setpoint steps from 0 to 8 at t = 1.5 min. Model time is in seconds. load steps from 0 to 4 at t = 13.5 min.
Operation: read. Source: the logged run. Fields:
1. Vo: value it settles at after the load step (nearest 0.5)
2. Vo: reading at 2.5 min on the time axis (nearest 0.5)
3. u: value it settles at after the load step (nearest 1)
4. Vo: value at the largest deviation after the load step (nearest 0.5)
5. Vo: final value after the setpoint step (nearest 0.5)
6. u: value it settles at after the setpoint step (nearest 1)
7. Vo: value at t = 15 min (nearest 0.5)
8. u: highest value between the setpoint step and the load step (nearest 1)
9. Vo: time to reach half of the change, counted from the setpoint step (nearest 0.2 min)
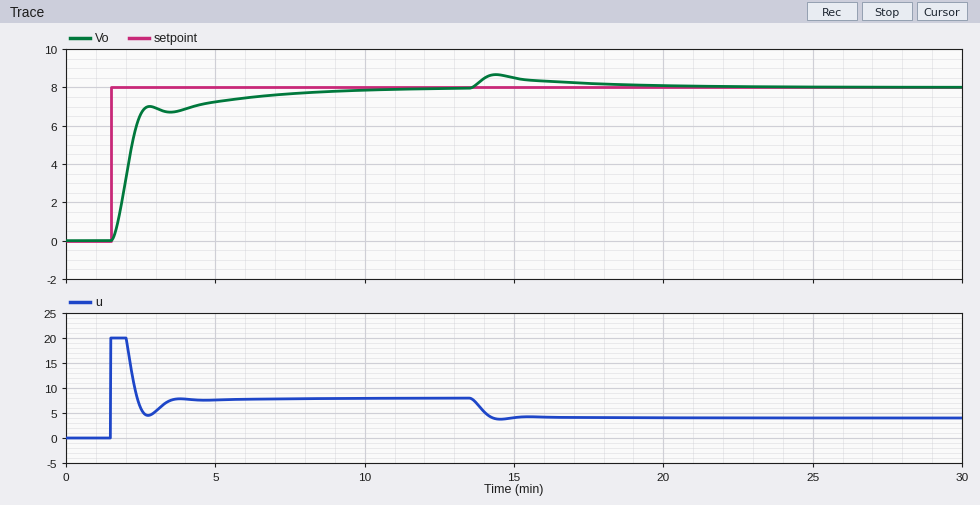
8.0
6.5
4
8.5
8.0
8
8.5
20
0.6 min
